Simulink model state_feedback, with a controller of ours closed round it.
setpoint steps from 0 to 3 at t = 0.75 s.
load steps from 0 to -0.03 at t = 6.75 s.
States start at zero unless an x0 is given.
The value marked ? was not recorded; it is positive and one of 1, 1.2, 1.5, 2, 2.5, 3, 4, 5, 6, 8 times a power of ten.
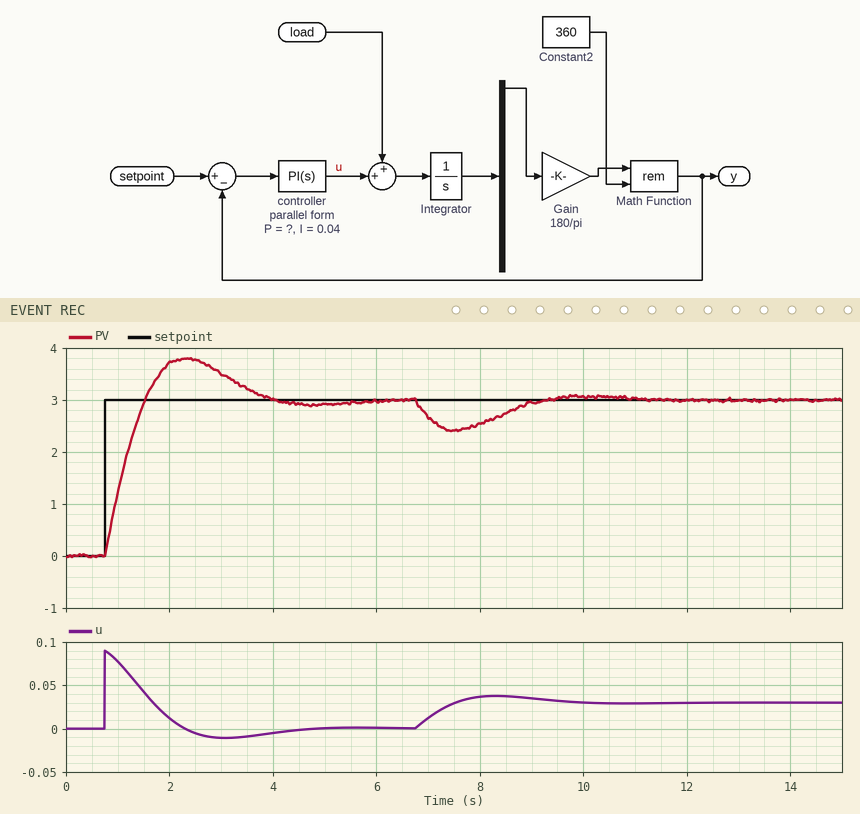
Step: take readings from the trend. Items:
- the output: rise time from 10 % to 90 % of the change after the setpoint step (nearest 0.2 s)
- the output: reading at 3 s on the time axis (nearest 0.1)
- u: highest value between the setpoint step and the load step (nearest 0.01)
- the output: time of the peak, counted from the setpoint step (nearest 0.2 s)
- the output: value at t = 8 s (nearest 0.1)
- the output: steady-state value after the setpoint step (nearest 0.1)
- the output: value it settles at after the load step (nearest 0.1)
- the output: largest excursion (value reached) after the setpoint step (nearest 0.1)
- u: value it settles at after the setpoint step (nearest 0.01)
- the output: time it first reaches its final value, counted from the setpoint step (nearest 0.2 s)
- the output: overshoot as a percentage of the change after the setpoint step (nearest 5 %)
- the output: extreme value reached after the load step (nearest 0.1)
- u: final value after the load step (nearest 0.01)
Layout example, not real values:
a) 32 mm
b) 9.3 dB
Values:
a) 0.6 s
b) 3.5
c) 0.09
d) 1.6 s
e) 2.5
f) 3.0
g) 3.0
h) 3.8
i) 0.00
j) 0.8 s
k) 25 %
l) 2.4
m) 0.03
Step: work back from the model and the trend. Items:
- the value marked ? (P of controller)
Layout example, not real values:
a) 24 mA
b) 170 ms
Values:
a) 0.03
